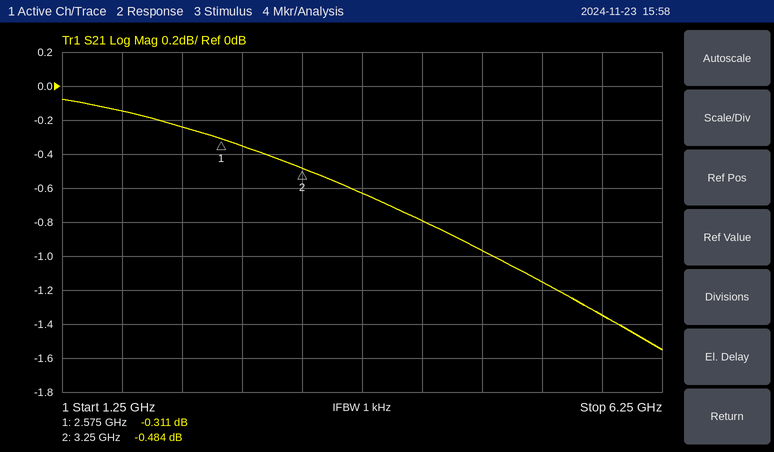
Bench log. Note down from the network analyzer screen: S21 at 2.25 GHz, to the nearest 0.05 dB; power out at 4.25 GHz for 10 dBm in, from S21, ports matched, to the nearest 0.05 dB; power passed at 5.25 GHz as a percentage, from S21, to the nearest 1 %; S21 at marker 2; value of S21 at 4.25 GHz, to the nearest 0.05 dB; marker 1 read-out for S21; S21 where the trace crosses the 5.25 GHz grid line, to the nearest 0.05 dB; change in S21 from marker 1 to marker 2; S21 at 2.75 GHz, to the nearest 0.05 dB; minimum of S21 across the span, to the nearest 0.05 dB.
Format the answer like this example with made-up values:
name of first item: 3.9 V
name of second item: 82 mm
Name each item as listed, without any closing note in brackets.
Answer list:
S21 at 2.25 GHz, to the nearest 0.05 dB: -0.25 dB
power out at 4.25 GHz for 10 dBm in, from S21, ports matched, to the nearest 0.05 dB: 9.20 dBm
power passed at 5.25 GHz as a percentage, from S21, to the nearest 1 %: 77 %
S21 at marker 2: -0.484 dB
value of S21 at 4.25 GHz, to the nearest 0.05 dB: -0.80 dB
marker 1 read-out for S21: -0.311 dB
S21 where the trace crosses the 5.25 GHz grid line, to the nearest 0.05 dB: -1.15 dB
change in S21 from marker 1 to marker 2: -0.173 dB
S21 at 2.75 GHz, to the nearest 0.05 dB: -0.35 dB
minimum of S21 across the span, to the nearest 0.05 dB: -1.55 dB
